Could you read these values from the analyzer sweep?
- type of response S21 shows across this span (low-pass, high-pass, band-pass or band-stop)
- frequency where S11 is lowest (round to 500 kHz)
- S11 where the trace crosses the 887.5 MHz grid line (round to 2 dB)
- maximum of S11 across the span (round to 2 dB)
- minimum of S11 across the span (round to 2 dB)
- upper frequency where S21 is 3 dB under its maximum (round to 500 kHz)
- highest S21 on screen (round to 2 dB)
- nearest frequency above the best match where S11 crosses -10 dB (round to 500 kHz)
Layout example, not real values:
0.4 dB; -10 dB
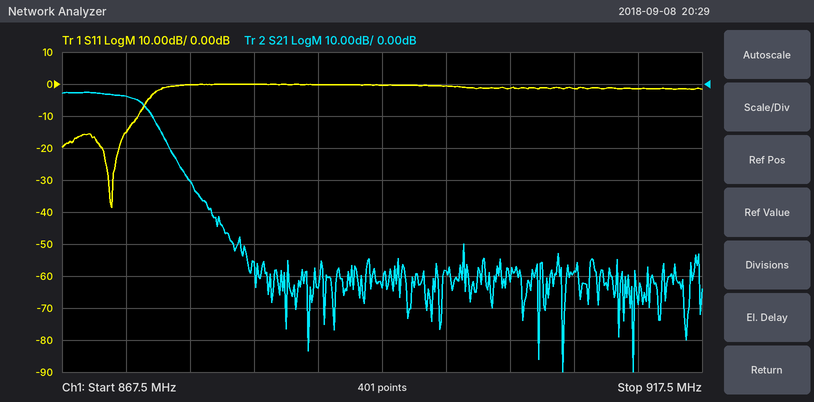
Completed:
low-pass; 871.5 MHz; 0 dB; 0 dB; -38 dB; 873.5 MHz; -2 dB; 873.5 MHz
